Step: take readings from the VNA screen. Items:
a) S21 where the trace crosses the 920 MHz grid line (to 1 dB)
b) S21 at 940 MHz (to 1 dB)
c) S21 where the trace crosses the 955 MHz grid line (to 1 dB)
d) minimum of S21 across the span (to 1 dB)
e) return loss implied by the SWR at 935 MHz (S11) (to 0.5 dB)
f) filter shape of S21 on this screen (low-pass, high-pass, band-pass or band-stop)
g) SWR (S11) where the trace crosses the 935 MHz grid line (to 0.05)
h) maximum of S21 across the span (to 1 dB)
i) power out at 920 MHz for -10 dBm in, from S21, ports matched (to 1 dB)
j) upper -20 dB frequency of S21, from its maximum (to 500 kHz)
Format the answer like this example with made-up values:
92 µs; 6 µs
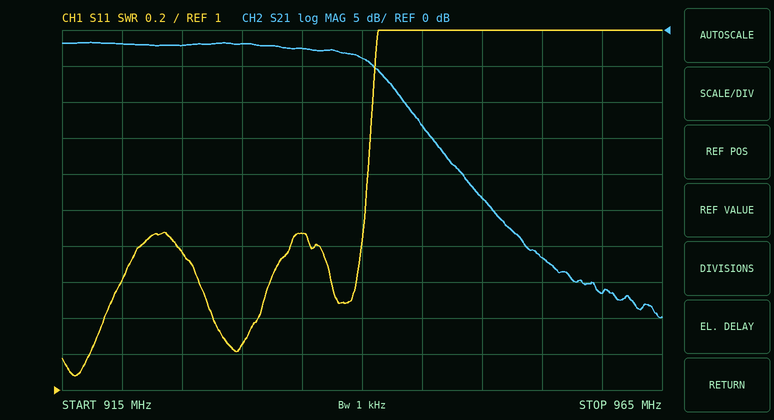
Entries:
-2 dB; -4 dB; -32 dB; -40 dB; 10.5 dB; low-pass; 1.85; -2 dB; -12 dBm; 949.0 MHz
